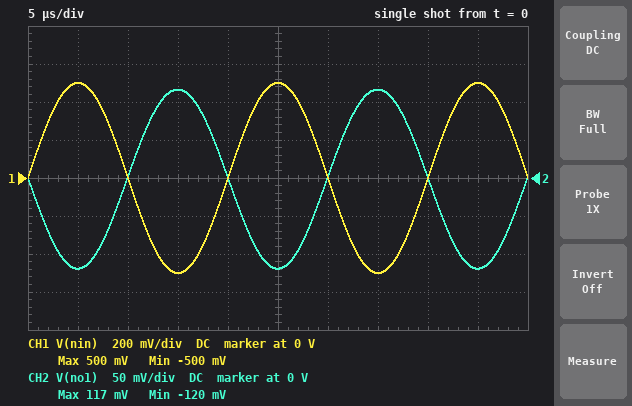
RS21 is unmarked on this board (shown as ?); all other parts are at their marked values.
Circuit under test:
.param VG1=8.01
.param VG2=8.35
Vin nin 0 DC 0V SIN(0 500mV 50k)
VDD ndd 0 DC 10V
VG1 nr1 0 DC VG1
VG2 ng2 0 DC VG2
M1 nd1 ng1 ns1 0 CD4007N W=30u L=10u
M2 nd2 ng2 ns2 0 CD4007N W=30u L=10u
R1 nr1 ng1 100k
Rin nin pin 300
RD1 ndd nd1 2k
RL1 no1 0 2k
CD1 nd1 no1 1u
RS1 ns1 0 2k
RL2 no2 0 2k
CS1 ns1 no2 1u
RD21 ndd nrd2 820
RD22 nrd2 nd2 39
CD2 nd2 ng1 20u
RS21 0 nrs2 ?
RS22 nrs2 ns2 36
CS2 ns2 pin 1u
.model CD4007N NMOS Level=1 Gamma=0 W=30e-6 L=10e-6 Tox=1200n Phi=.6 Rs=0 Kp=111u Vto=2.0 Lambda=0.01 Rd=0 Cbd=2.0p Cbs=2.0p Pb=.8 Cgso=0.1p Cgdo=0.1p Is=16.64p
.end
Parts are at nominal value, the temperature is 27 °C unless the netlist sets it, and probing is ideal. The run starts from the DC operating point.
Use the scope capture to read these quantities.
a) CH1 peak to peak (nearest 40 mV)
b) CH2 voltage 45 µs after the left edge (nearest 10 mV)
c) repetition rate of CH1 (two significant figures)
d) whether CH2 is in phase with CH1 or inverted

1.00 V
-120 mV
50 kHz
inverted
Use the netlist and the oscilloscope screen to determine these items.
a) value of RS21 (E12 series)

180 Ω
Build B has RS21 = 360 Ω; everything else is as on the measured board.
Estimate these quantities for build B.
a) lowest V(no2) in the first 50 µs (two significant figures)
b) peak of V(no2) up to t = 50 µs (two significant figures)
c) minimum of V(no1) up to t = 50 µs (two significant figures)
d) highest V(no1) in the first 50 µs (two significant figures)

-160 mV
150 mV
-150 mV
160 mV
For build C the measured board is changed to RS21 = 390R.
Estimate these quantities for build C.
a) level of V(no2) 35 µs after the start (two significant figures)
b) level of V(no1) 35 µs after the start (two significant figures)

-160 mV
160 mV
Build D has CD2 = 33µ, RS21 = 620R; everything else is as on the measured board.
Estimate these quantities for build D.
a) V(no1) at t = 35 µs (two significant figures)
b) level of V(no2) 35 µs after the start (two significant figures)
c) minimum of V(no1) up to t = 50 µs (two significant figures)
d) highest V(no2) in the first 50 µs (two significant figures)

170 mV
-170 mV
-160 mV
160 mV
